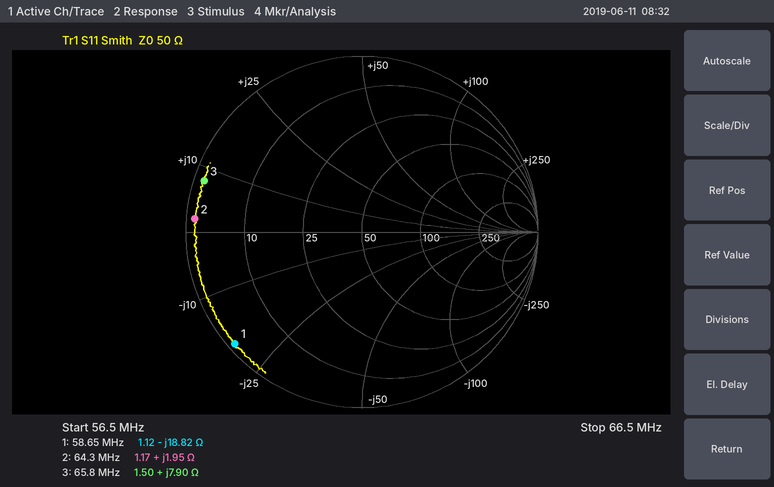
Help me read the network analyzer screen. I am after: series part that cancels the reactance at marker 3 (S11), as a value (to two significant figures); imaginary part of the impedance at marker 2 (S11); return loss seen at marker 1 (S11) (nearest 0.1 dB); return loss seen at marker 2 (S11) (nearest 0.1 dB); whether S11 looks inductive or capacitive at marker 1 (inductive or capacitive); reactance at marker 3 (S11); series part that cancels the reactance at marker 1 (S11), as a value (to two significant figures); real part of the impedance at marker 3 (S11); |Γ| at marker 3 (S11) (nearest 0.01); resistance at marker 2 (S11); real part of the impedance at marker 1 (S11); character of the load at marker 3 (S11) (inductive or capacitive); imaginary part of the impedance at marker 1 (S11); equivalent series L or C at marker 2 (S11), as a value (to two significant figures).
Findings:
310 pF
+1.95 Ω
0.3 dB
0.4 dB
capacitive
+7.90 Ω
51 nH
1.50 Ω
0.94
1.17 Ω
1.12 Ω
inductive
-18.82 Ω
4.8 nH
